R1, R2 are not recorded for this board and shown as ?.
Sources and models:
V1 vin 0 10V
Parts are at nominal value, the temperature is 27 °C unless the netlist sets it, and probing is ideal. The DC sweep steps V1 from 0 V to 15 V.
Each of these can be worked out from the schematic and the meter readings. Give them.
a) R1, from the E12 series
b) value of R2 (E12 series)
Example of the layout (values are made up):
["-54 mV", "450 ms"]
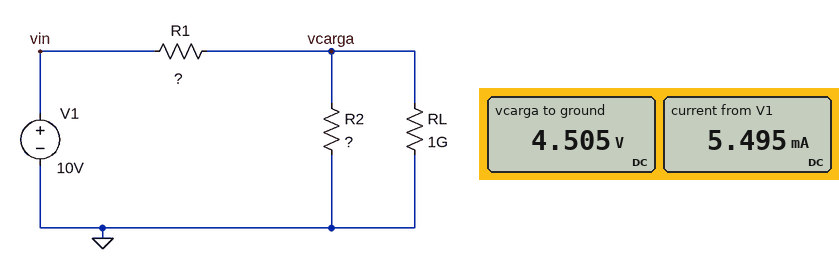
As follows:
["1 kΩ", "820 Ω"]
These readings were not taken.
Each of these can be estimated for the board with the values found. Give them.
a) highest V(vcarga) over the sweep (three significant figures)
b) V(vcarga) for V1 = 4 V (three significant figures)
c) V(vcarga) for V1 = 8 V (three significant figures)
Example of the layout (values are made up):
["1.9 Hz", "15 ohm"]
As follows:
["6.76 V", "1.80 V", "3.60 V"]
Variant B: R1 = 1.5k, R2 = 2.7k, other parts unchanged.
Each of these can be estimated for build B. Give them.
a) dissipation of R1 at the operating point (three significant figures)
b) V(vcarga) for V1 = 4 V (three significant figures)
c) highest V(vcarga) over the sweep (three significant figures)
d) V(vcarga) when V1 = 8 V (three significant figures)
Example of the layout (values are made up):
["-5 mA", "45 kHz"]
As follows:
["8.50 mW", "2.57 V", "9.64 V", "5.14 V"]
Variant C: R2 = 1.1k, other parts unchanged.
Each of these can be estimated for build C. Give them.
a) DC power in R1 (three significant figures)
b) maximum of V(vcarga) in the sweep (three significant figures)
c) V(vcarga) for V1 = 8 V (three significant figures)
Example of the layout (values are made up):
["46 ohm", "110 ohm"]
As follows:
["22.7 mW", "7.86 V", "4.19 V"]
